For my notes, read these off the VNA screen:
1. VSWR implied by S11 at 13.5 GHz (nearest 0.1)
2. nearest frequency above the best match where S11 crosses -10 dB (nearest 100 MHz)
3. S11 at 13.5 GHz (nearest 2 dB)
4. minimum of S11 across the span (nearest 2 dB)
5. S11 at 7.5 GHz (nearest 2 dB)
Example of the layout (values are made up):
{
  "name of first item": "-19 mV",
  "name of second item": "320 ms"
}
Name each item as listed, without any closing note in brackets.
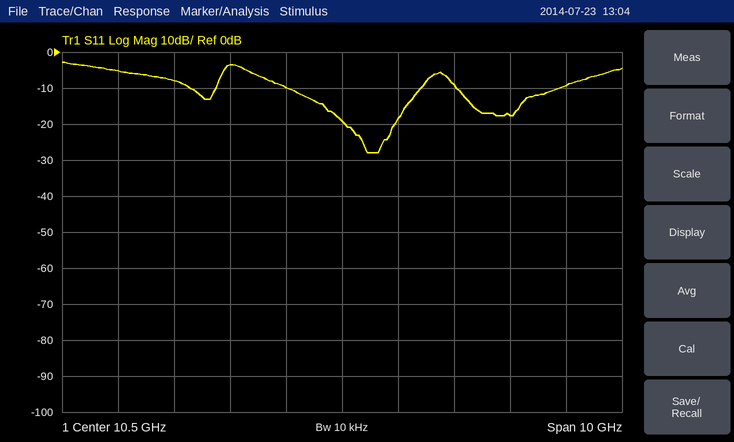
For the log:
{
  "VSWR implied by S11 at 13.5 GHz": "1.3",
  "nearest frequency above the best match where S11 crosses -10 dB": "11.9 GHz",
  "S11 at 13.5 GHz": "-18 dB",
  "minimum of S11 across the span": "-28 dB",
  "S11 at 7.5 GHz": "-8 dB"
}
